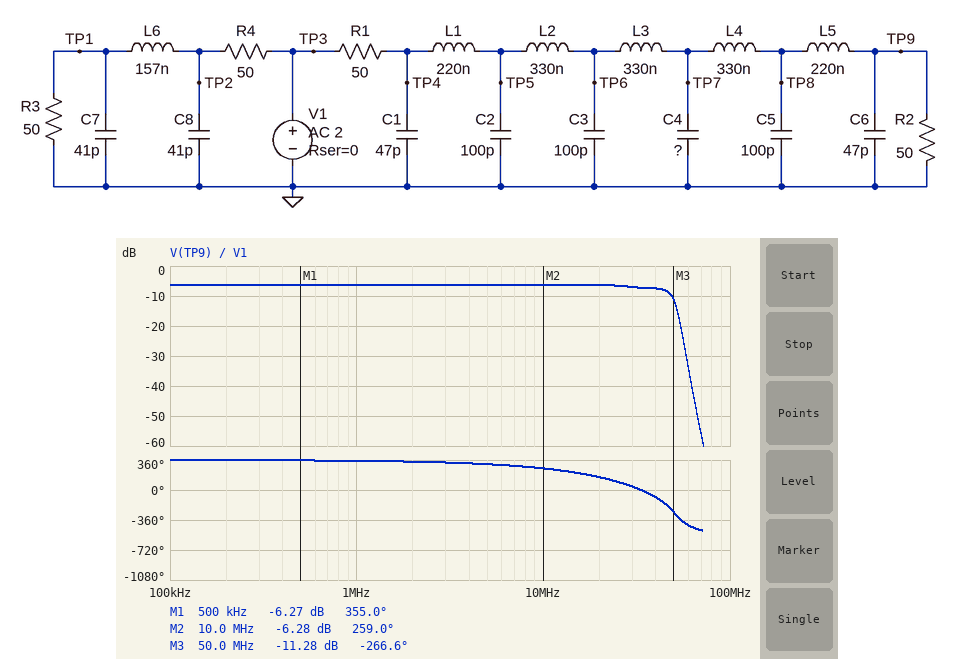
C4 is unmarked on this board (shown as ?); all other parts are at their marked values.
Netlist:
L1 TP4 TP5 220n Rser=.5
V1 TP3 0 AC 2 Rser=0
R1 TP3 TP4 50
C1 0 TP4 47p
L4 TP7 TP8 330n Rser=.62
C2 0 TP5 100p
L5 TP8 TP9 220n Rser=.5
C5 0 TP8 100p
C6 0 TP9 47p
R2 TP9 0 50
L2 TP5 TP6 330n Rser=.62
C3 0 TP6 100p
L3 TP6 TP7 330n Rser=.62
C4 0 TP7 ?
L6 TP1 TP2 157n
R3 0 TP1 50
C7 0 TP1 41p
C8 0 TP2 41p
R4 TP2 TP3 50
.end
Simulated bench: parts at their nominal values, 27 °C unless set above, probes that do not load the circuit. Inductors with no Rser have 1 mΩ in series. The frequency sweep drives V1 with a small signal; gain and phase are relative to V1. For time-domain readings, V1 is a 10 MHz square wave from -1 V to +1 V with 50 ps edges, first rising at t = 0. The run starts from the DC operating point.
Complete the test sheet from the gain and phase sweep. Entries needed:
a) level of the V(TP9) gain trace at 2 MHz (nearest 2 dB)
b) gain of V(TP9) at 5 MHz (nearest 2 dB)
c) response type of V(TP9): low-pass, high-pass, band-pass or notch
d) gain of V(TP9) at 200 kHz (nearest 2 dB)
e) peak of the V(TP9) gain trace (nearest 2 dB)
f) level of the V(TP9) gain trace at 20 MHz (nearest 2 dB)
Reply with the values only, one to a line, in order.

-6 dB
-6 dB
low-pass
-6 dB
-6 dB
-6 dB
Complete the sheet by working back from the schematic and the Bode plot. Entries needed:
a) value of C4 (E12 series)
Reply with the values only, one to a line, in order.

150 pF
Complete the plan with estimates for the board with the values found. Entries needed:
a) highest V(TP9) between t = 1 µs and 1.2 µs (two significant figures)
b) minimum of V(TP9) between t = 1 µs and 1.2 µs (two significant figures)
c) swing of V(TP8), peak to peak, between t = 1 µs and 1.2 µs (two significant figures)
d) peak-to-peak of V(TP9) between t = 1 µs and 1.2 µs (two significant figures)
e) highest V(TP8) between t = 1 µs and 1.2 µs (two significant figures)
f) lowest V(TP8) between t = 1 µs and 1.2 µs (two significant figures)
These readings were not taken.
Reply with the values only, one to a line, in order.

670 mV
-670 mV
1.4 V
1.3 V
700 mV
-700 mV
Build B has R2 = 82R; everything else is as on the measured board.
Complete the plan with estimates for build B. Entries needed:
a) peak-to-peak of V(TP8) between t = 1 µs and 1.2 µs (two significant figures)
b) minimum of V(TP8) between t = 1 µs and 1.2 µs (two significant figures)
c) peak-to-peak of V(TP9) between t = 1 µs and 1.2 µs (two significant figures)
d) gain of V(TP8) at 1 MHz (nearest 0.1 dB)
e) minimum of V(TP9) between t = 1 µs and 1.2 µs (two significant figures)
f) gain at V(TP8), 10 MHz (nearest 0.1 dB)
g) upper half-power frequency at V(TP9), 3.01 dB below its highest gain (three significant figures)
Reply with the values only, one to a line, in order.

1.5 V
-730 mV
1.7 V
-4.3 dB
-840 mV
-4.5 dB
45.0 MHz
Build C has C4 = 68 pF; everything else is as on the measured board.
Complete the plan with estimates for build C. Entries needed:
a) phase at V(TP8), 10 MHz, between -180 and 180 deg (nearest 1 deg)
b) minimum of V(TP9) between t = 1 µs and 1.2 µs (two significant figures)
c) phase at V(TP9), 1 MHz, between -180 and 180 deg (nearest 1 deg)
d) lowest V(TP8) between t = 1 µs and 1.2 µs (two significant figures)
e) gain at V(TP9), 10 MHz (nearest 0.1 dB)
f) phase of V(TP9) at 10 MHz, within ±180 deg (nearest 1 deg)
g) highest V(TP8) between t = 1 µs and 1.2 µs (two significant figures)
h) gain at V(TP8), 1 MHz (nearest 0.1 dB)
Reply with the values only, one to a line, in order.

-77 deg
-650 mV
-9 deg
-680 mV
-6.4 dB
-93 deg
680 mV
-6.2 dB
